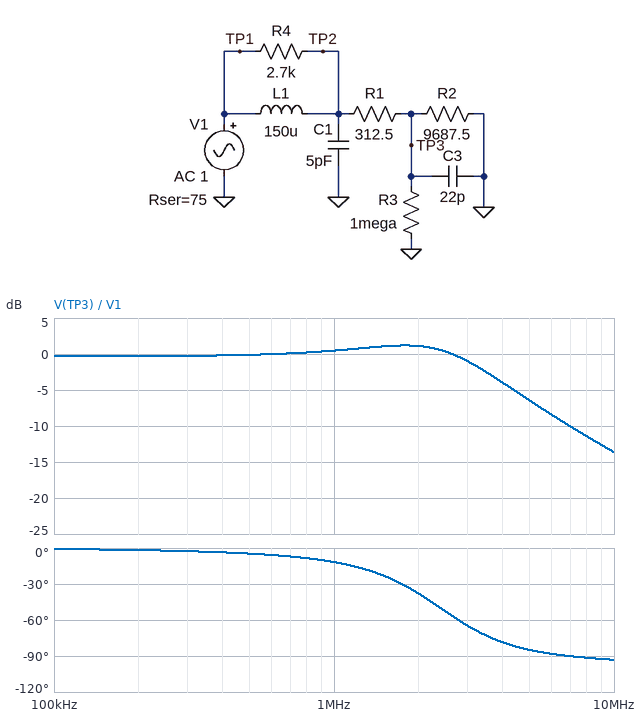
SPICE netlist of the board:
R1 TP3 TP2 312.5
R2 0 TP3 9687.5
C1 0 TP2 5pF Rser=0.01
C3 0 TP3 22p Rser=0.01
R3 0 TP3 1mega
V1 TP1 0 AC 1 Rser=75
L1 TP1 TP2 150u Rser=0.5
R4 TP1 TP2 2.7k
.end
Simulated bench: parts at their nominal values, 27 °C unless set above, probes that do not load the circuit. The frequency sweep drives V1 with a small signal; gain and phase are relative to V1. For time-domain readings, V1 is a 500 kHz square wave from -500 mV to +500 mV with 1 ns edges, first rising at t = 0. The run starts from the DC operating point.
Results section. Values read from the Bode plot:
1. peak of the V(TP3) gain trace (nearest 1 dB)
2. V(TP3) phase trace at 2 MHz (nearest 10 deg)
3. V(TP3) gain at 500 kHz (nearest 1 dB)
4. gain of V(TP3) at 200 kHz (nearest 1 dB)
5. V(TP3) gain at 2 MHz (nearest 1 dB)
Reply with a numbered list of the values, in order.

1. 1 dB
2. -40 deg
3. 0 dB
4. 0 dB
5. 1 dB
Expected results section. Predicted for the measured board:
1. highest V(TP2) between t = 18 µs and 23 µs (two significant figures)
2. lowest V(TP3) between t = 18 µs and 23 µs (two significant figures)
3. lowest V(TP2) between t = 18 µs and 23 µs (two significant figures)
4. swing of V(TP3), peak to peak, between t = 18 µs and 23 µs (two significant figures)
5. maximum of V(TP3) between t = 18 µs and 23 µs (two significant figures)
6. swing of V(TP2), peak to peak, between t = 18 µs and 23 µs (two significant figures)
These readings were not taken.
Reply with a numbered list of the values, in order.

1. 660 mV
2. -640 mV
3. -660 mV
4. 1.3 V
5. 640 mV
6. 1.3 V
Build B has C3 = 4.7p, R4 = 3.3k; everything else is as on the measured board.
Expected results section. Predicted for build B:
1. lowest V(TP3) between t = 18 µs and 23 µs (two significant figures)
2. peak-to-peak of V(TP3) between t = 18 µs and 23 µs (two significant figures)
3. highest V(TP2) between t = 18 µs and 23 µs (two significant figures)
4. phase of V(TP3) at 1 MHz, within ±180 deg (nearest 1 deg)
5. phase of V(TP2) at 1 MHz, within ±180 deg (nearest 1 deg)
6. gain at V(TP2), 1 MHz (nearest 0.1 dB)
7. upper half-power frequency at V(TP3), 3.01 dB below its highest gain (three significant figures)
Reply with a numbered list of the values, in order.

1. -550 mV
2. 1.1 V
3. 570 mV
4. -7 deg
5. -6 deg
6. 0.1 dB
7. 6.22 MHz
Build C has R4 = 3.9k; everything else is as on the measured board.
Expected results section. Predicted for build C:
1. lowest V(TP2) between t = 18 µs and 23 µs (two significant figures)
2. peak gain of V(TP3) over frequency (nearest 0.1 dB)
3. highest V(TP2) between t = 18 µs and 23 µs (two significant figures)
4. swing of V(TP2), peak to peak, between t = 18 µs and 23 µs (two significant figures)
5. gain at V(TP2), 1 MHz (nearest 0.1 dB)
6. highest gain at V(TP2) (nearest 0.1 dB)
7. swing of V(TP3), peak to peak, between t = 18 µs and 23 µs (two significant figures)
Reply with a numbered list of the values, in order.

1. -730 mV
2. 2.1 dB
3. 730 mV
4. 1.5 V
5. 0.9 dB
6. 2.4 dB
7. 1.4 V
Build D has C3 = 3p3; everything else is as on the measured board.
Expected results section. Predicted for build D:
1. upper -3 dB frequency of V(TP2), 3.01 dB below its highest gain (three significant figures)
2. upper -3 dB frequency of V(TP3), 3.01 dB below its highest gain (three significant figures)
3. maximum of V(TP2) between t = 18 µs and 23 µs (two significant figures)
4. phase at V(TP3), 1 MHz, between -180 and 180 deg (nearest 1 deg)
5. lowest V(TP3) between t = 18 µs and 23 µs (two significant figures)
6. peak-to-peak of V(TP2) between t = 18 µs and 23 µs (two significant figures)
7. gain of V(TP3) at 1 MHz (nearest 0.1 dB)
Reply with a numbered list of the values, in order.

1. 7.77 MHz
2. 7.76 MHz
3. 530 mV
4. -6 deg
5. -510 mV
6. 1.1 V
7. -0.3 dB
